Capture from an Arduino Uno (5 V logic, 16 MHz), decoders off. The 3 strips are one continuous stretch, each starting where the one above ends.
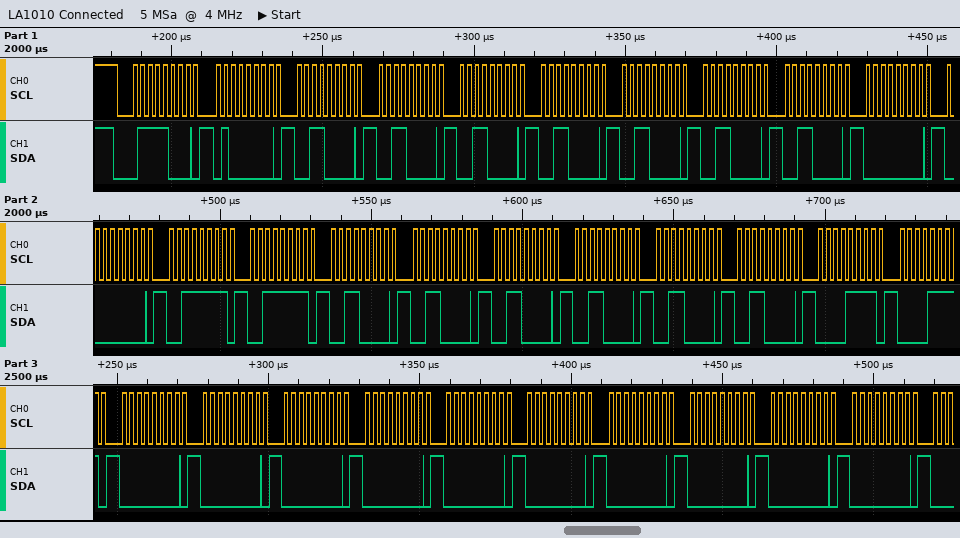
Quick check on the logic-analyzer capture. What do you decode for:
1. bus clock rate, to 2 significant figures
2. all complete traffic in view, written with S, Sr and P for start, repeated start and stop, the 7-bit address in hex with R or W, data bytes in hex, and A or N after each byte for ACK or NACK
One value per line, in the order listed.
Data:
400 kHz
S 3CW A 40 A 30 A 30 A 30 A 30 A 30 A 30 A 30 A 00 A 00 A 3F A 3F A 30 A 30 A 30 A 30 A 30 A 30 A 0F A 0F A 00 A 00 A 00 A 00 A 00 A 00 A 00 A 00 A 00 A 00 A
